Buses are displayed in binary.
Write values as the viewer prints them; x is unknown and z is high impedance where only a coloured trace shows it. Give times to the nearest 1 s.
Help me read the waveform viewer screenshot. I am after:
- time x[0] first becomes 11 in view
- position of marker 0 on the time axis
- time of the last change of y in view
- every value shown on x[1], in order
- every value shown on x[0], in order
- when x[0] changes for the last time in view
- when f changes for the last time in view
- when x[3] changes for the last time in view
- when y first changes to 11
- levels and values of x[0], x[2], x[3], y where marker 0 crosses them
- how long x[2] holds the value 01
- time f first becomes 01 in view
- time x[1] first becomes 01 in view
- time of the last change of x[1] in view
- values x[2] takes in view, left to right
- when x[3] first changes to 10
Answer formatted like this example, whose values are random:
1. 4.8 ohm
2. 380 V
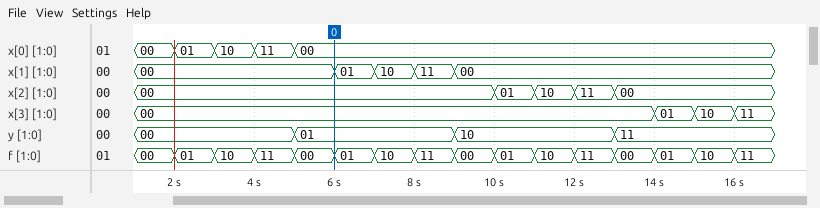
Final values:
1. 4 s
2. 6 s
3. 13 s
4. 00, 01, 10, 11, 00
5. 00, 01, 10, 11, 00
6. 5 s
7. 16 s
8. 16 s
9. 13 s
10. x[0]=00, x[2]=00, x[3]=00, y=01
11. 1 s
12. 2 s
13. 6 s
14. 9 s
15. 00, 01, 10, 11, 00
16. 15 s
